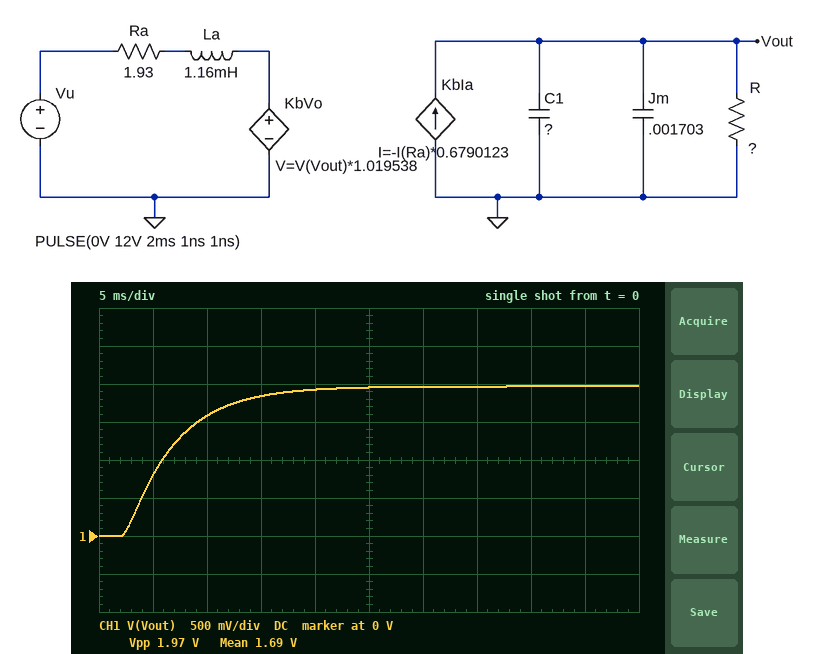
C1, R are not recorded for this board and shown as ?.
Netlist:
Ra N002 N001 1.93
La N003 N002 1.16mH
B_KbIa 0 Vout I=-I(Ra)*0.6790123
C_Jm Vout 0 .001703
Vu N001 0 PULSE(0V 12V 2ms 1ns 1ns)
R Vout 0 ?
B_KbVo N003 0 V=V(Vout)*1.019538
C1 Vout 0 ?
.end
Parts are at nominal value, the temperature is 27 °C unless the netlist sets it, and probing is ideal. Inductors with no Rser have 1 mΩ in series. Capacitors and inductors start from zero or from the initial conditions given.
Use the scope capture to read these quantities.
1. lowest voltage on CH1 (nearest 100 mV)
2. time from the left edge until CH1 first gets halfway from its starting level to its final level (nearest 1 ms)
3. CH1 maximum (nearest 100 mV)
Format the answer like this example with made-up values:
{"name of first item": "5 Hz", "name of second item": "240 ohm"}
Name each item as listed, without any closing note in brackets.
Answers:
{"lowest voltage on CH1": "0 V", "time from the left edge until CH1 first gets halfway from its starting level to its final level": "6 ms", "CH1 maximum": "2.0 V"}
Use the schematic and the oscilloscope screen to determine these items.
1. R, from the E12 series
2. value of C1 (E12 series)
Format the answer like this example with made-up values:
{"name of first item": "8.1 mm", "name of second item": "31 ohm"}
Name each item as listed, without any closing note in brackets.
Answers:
{"R, from the E12 series": "0.56 Ω", "value of C1": "8.2 mF"}
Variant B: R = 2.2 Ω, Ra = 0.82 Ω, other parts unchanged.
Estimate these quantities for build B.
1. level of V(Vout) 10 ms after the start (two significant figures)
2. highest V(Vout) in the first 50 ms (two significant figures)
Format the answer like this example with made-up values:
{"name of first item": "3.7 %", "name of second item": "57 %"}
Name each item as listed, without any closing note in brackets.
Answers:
{"level of V(Vout) 10 ms after the start": "4.7 V", "highest V(Vout) in the first 50 ms": "7.6 V"}
